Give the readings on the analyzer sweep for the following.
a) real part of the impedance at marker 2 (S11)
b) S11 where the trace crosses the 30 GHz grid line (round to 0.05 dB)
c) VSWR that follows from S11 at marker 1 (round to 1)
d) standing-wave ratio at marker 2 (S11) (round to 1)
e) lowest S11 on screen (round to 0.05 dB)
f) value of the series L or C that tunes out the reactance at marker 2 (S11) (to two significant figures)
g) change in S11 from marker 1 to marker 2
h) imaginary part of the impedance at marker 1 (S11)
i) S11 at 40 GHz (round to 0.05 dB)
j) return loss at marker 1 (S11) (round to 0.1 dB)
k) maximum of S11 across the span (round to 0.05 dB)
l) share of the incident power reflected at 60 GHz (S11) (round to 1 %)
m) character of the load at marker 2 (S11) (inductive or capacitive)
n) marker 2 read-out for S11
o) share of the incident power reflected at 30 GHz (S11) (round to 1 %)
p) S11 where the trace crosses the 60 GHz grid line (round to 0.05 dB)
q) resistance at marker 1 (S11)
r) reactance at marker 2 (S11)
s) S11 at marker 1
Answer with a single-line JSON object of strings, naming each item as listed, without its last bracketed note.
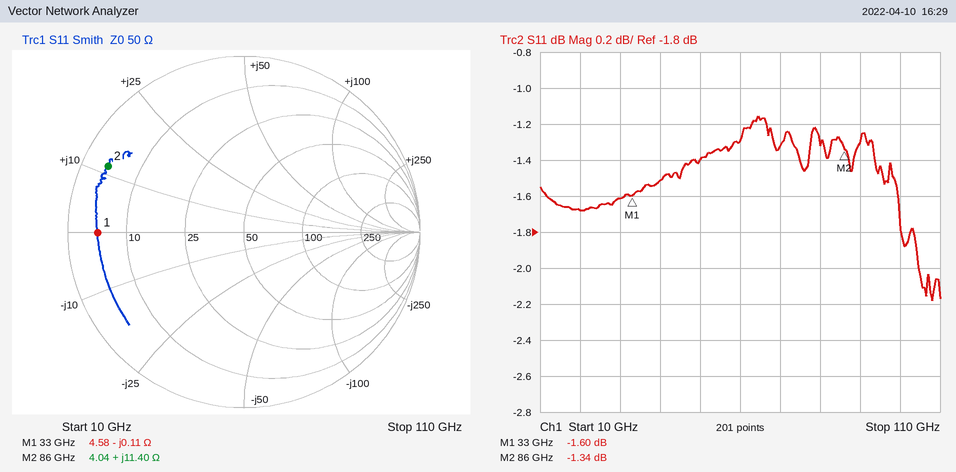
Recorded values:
{"real part of the impedance at marker 2": "4.04 Ω", "S11 where the trace crosses the 30 GHz grid line": "-1.60 dB", "VSWR that follows from S11 at marker 1": "11", "standing-wave ratio at marker 2 (S11)": "13", "lowest S11 on screen": "-2.20 dB", "value of the series L or C that tunes out the reactance at marker 2 (S11)": "160 fF", "change in S11 from marker 1 to marker 2": "0.26 dB", "imaginary part of the impedance at marker 1": "-0.11 Ω", "S11 at 40 GHz": "-1.50 dB", "return loss at marker 1 (S11)": "1.6 dB", "maximum of S11 across the span": "-1.15 dB", "share of the incident power reflected at 60 GHz (S11)": "74 %", "character of the load at marker 2 (S11)": "inductive", "marker 2 read-out for S11": "-1.34 dB", "share of the incident power reflected at 30 GHz (S11)": "69 %", "S11 where the trace crosses the 60 GHz grid line": "-1.30 dB", "resistance at marker 1": "4.58 Ω", "reactance at marker 2": "+11.40 Ω", "S11 at marker 1": "-1.60 dB"}
